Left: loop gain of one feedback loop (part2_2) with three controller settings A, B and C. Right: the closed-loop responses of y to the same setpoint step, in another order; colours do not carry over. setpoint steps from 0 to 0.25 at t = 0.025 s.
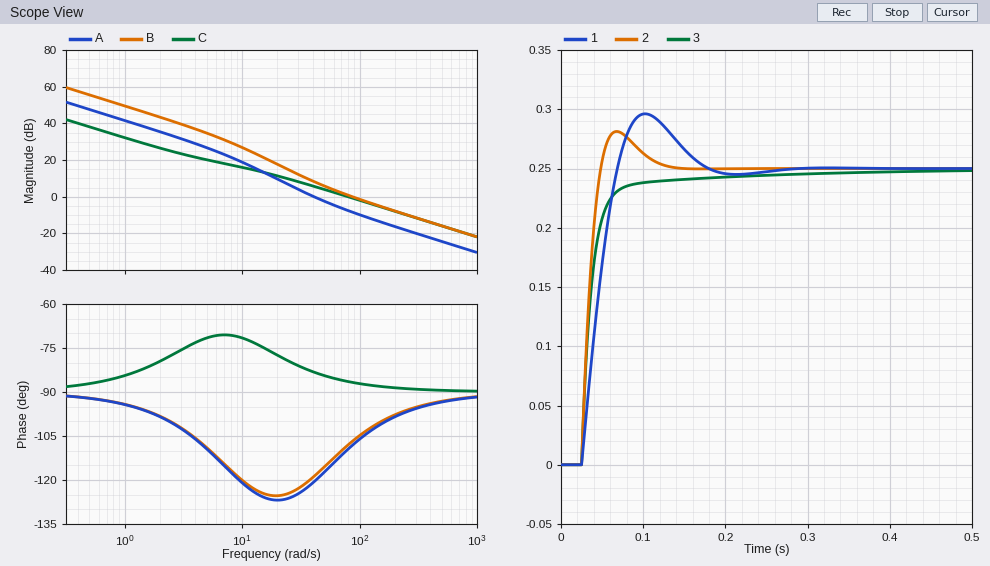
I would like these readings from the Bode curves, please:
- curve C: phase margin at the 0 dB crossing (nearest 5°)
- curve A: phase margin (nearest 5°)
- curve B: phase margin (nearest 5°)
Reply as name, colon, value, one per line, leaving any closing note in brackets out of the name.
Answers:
curve C: phase margin at the 0 dB crossing: 95°
curve A: phase margin: 60°
curve B: phase margin: 75°
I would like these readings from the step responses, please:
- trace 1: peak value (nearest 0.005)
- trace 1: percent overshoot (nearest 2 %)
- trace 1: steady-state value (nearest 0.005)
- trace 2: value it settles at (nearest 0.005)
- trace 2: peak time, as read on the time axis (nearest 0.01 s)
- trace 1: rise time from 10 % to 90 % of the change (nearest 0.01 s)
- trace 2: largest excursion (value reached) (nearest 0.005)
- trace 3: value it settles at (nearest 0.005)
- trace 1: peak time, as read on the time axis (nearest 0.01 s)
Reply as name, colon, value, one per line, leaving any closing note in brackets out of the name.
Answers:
trace 1: peak value: 0.295
trace 1: percent overshoot: 18 %
trace 1: steady-state value: 0.250
trace 2: value it settles at: 0.250
trace 2: peak time, as read on the time axis: 0.07 s
trace 1: rise time from 10 % to 90 % of the change: 0.03 s
trace 2: largest excursion (value reached): 0.280
trace 3: value it settles at: 0.250
trace 1: peak time, as read on the time axis: 0.10 s
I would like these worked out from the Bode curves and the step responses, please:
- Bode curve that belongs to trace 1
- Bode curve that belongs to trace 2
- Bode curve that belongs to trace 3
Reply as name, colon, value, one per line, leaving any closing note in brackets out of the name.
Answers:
Bode curve that belongs to trace 1: A
Bode curve that belongs to trace 2: B
Bode curve that belongs to trace 3: C
